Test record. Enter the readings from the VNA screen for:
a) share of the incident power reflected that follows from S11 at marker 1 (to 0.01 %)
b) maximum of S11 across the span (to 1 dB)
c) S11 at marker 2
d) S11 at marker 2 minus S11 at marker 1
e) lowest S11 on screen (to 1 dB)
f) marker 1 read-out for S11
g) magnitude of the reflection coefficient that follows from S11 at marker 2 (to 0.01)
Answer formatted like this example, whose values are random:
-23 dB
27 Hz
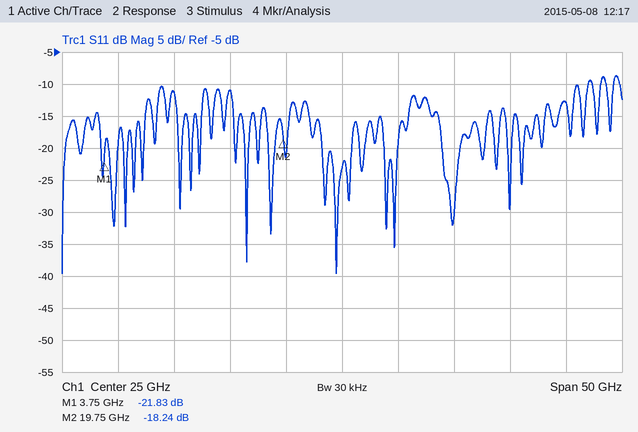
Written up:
0.66 %
-9 dB
-18.24 dB
3.59 dB
-40 dB
-21.83 dB
0.12
